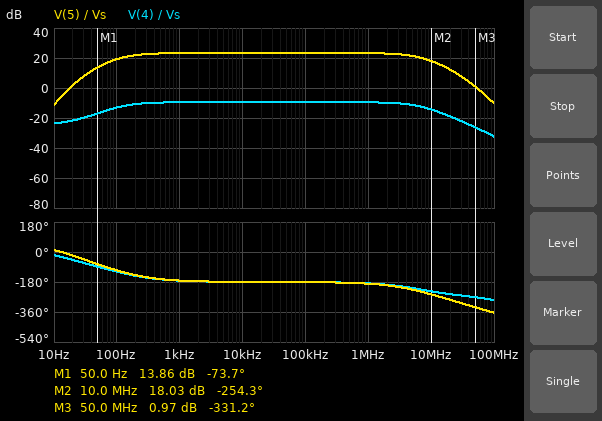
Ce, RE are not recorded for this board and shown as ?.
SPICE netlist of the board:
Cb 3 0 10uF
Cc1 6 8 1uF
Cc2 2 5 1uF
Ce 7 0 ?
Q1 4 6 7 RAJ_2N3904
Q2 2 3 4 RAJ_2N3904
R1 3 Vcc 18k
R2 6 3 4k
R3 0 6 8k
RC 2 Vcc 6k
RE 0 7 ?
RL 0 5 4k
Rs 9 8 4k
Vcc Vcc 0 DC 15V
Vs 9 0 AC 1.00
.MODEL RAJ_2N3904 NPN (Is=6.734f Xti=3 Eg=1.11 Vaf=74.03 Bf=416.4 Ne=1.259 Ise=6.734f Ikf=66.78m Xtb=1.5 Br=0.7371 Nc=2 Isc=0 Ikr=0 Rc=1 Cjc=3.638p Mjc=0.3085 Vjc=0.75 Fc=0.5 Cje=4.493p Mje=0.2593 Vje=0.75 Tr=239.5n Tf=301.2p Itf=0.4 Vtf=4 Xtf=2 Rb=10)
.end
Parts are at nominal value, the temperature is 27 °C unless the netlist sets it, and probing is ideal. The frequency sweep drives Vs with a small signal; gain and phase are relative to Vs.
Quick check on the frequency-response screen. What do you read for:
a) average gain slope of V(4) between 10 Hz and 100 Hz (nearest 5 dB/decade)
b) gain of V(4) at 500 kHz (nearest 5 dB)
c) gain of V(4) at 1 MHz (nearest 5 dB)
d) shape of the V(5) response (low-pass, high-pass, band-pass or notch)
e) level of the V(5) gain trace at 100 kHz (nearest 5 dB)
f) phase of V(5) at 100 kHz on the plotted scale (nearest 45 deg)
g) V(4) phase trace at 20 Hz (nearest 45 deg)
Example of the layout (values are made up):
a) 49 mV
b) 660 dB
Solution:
a) 10 dB/decade
b) -10 dB
c) -10 dB
d) band-pass
e) 25 dB
f) -180 deg
g) -45 deg
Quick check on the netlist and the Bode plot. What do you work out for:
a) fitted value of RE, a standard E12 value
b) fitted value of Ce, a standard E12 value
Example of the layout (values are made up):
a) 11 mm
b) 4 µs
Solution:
a) 6.8 kΩ
b) 22 µF
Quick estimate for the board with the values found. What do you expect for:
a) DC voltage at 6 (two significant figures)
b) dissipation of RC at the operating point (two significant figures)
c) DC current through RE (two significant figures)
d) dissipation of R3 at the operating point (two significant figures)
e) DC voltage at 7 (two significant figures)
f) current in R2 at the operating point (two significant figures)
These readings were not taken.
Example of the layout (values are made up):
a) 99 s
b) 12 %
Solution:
a) 4.0 V
b) 1.4 mW
c) 490 µA
d) 2.0 mW
e) 3.3 V
f) 500 µA
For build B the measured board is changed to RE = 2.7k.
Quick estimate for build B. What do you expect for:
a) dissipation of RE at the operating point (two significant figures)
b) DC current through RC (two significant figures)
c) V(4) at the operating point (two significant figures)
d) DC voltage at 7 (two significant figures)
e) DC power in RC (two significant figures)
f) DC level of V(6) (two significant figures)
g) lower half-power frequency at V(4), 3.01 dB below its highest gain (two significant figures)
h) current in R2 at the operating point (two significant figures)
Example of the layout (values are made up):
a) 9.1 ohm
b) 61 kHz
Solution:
a) 3.9 mW
b) 1.2 mA
c) 5.2 V
d) 3.2 V
e) 8.4 mW
f) 3.9 V
g) 230 Hz
h) 500 µA
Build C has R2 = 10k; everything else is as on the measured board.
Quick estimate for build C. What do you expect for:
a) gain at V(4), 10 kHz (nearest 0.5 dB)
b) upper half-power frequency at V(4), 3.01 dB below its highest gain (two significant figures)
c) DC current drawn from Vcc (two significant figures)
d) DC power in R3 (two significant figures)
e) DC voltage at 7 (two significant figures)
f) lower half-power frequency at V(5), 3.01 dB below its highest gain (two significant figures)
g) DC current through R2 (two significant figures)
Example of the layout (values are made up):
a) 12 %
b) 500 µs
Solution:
a) -7.0 dB
b) 6.1 MHz
c) 800 µA
d) 1.4 mW
e) 2.7 V
f) 100 Hz
g) 420 µA
